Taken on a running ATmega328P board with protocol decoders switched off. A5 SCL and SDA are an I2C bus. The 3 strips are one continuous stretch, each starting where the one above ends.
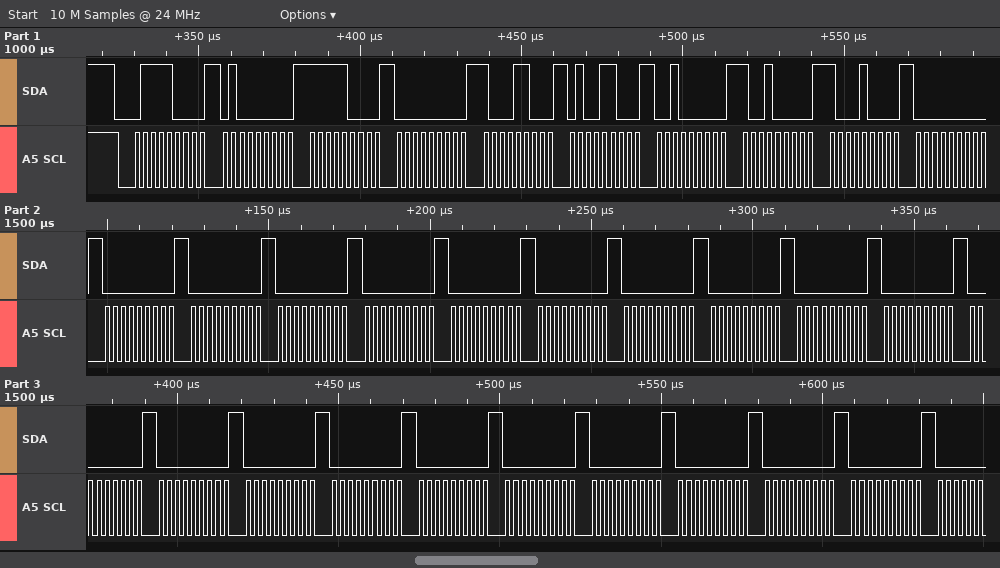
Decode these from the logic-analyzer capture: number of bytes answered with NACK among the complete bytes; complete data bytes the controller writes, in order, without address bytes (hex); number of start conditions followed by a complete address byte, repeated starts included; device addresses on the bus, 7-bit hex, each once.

0
40 F8 00 8C 4C 20 90 88 00 00 00 00 00 00 00 00 00 00 00 00 00 00 00 00 00 00 00 00 00
1
0x3C
